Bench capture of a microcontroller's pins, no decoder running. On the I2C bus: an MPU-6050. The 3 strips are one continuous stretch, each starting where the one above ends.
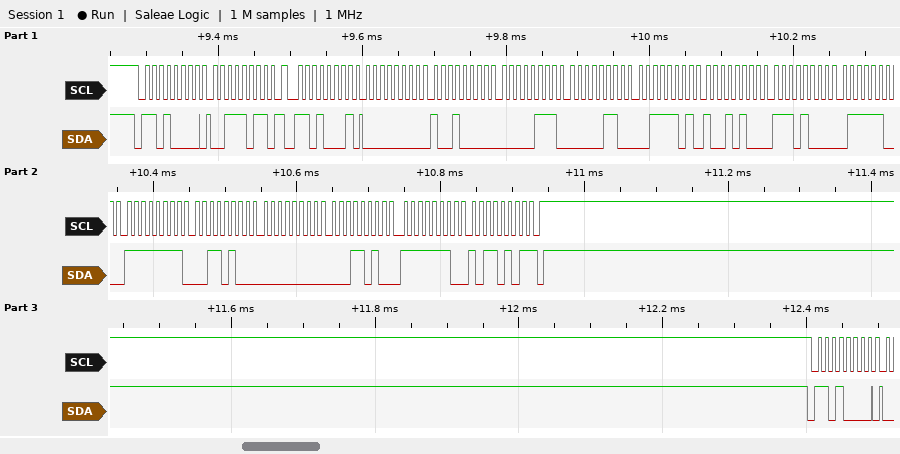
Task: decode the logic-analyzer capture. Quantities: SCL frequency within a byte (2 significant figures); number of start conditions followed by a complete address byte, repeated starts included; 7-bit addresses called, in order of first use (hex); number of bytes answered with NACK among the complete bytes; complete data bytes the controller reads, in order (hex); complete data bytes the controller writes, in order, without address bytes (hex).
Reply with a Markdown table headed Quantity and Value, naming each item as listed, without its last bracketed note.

| Quantity | Value |
|---|---|
| SCL frequency within a byte | 100 kHz |
| number of start conditions followed by a complete address byte, repeated starts included | 3 |
| 7-bit addresses called, in order of first use | 0x68 |
| number of bytes answered with NACK among the complete bytes | 1 |
| complete data bytes the controller reads, in order | 00 90 07 06 3D 94 E8 7C FF 34 00 1A FE B5 |
| complete data bytes the controller writes, in order, without address bytes | 3B |
